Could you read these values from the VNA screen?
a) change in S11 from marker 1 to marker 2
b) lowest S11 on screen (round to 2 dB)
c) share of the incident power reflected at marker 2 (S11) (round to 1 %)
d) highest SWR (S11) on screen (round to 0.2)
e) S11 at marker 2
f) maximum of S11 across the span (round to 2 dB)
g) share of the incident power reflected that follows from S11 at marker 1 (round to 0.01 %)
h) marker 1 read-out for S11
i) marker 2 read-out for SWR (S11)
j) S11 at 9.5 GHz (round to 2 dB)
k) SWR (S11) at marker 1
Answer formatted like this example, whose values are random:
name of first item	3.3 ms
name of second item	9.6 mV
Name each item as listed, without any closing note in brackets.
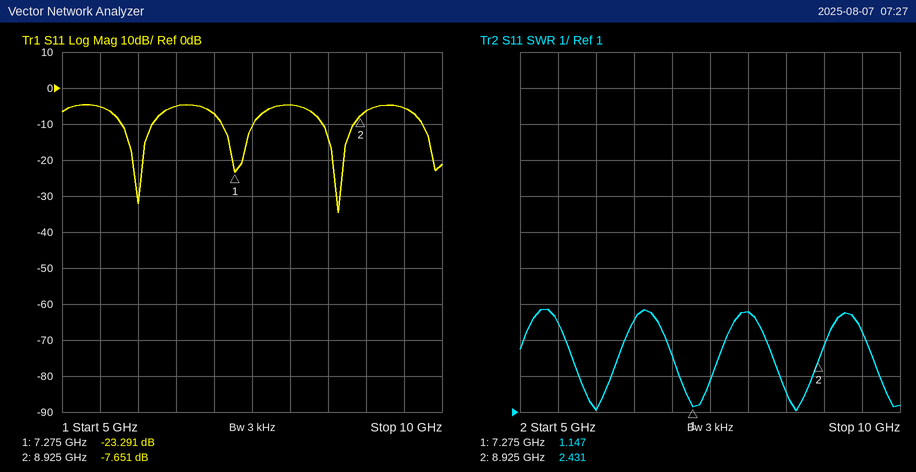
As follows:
change in S11 from marker 1 to marker 2	15.640 dB
lowest S11 on screen	-34 dB
share of the incident power reflected at marker 2 (S11)	17 %
highest SWR (S11) on screen	3.8
S11 at marker 2	-7.651 dB
maximum of S11 across the span	-4 dB
share of the incident power reflected that follows from S11 at marker 1	0.47 %
marker 1 read-out for S11	-23.291 dB
marker 2 read-out for SWR	2.431
S11 at 9.5 GHz	-6 dB
SWR (S11) at marker 1	1.147
